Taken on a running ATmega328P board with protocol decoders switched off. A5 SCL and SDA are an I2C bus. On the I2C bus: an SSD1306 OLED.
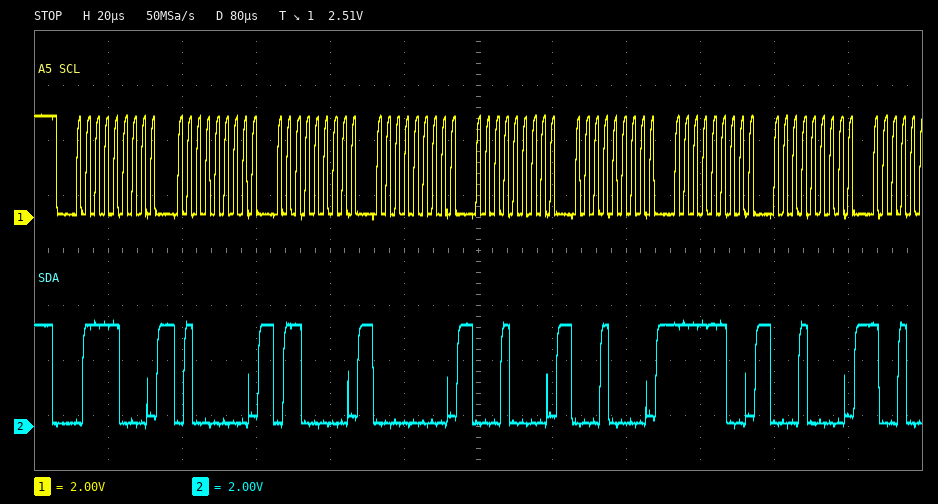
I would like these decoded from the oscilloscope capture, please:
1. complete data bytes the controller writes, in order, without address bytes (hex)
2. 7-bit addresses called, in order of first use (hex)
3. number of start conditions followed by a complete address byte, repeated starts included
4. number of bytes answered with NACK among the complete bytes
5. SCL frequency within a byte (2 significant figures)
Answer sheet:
40 60 00 10 10 FC 10
0x3C
1
0
400 kHz
